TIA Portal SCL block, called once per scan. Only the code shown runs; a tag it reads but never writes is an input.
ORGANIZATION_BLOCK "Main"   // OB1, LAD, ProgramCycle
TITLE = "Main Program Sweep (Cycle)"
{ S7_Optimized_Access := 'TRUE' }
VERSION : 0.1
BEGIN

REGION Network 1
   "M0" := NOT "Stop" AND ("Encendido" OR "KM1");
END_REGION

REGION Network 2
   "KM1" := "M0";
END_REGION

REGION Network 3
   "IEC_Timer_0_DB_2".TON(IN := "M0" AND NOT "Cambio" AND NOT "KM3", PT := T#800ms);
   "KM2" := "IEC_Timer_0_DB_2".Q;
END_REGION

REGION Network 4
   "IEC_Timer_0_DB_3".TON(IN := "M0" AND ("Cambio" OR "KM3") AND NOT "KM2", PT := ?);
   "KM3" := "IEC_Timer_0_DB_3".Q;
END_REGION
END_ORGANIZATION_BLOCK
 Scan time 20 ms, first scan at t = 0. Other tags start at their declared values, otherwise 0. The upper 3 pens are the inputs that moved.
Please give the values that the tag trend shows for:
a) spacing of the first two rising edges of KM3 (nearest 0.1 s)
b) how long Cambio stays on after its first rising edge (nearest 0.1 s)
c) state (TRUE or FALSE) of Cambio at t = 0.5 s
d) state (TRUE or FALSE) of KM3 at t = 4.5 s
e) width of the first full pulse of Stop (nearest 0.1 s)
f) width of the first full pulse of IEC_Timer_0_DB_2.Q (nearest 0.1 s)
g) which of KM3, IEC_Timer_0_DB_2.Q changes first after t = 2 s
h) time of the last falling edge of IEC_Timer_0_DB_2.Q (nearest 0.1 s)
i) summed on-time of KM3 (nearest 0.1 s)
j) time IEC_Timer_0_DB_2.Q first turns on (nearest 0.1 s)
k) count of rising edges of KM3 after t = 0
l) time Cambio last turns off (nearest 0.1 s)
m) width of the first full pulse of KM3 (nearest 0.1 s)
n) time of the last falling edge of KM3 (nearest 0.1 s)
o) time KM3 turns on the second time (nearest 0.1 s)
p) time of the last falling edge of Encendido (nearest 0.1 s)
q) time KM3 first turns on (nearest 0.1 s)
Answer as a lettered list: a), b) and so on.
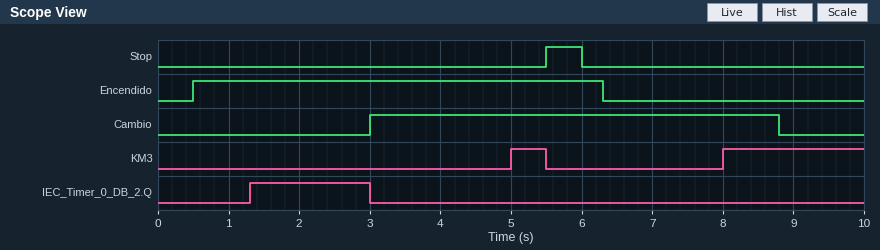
a) 3.0 s
b) 5.8 s
c) FALSE
d) FALSE
e) 0.5 s
f) 1.7 s
g) IEC_Timer_0_DB_2.Q
h) 3.0 s
i) 2.5 s
j) 1.3 s
k) 2
l) 8.8 s
m) 0.5 s
n) 5.5 s
o) 8.0 s
p) 6.3 s
q) 5.0 s
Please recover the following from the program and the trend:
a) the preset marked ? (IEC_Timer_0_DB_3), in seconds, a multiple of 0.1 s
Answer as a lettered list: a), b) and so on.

a) 2.0 s
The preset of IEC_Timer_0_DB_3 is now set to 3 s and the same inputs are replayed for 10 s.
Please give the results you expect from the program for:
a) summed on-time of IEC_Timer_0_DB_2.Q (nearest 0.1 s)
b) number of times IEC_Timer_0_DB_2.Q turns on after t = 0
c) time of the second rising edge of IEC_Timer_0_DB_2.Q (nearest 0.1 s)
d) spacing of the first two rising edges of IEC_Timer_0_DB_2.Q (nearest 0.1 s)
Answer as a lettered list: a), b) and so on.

a) 2.1 s
b) 2
c) 9.6 s
d) 8.3 s
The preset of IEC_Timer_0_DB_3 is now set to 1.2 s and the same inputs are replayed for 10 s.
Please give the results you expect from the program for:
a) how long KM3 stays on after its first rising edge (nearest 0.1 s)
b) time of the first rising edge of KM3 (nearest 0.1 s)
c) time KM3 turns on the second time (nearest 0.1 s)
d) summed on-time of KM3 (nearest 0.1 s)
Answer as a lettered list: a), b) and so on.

a) 1.3 s
b) 4.2 s
c) 7.2 s
d) 4.1 s
